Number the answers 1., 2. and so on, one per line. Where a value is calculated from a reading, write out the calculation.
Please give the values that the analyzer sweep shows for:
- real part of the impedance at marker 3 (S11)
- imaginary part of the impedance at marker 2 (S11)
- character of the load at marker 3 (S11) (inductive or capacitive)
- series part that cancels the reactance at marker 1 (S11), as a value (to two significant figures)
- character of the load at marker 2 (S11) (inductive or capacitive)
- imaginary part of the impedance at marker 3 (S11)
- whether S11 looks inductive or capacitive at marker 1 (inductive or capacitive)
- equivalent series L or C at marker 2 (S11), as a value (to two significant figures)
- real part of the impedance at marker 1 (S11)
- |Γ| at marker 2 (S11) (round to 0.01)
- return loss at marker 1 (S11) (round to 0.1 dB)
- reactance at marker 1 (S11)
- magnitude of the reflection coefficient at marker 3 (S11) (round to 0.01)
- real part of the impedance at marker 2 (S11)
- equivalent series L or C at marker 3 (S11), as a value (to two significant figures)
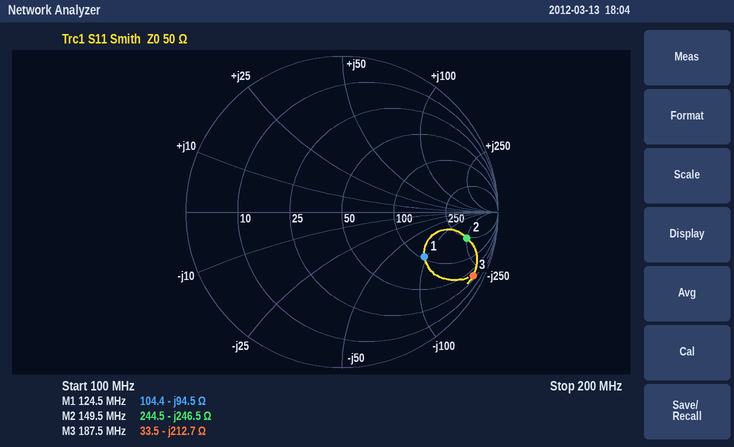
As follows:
1. 33.5 Ω
2. -246.5 Ω
3. capacitive
4. L = 94.5 Ω/(2π × 124.5 MHz) ≈ 121 nH, so 120 nH to two significant figures
5. capacitive
6. -212.7 Ω
7. capacitive
8. C = 1/(2π × 149.5 MHz × 246.5 Ω) ≈ 4.3 pF
9. 104.4 Ω
10. 0.82
11. 4.4 dB
12. -94.5 Ω
13. 0.93
14. 244.5 Ω
15. C = 1/(2π × 187.5 MHz × 212.7 Ω) ≈ 4.0 pF
